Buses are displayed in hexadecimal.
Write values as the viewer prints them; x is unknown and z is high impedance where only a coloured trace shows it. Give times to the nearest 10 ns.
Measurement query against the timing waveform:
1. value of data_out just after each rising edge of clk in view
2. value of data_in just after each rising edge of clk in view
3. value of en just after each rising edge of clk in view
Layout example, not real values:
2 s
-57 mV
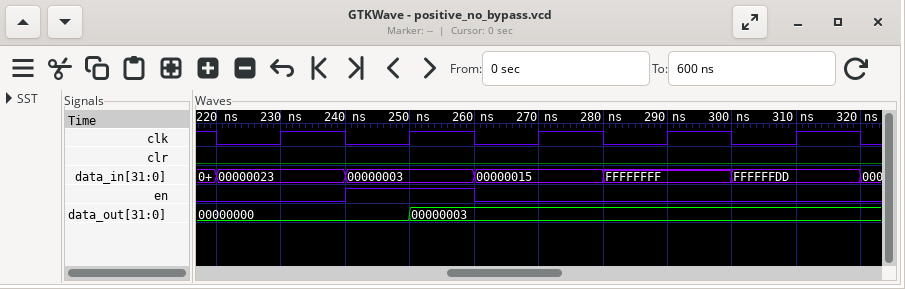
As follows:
00000000, 00000003, 00000003, 00000003, 00000003
00000023, 00000003, 00000015, FFFFFFFF, FFFFFFDD
0 1 0 0 0
